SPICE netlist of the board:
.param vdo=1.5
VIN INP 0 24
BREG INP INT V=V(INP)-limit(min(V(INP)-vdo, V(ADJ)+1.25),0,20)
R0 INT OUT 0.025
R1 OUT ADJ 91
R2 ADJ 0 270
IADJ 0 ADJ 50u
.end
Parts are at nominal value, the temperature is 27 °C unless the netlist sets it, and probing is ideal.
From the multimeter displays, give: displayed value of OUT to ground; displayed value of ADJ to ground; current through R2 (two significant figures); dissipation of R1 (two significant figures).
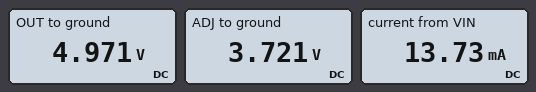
4.971 V
3.721 V
14 mA
17 mW
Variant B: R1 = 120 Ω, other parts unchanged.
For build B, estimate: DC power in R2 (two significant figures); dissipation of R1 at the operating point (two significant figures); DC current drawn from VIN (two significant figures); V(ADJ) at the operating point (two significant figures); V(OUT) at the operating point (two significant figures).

30 mW
13 mW
10 mA
2.8 V
4.1 V
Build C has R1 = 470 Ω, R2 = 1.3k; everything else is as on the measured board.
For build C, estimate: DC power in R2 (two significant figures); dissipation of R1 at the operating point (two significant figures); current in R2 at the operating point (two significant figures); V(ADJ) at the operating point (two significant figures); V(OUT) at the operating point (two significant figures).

9.5 mW
3.3 mW
2.7 mA
3.5 V
4.8 V
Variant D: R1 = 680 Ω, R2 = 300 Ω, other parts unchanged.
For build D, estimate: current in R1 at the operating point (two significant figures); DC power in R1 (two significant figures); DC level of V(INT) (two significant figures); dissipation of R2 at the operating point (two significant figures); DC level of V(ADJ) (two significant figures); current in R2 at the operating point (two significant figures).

1.8 mA
2.3 mW
1.8 V
1.1 mW
570 mV
1.9 mA
